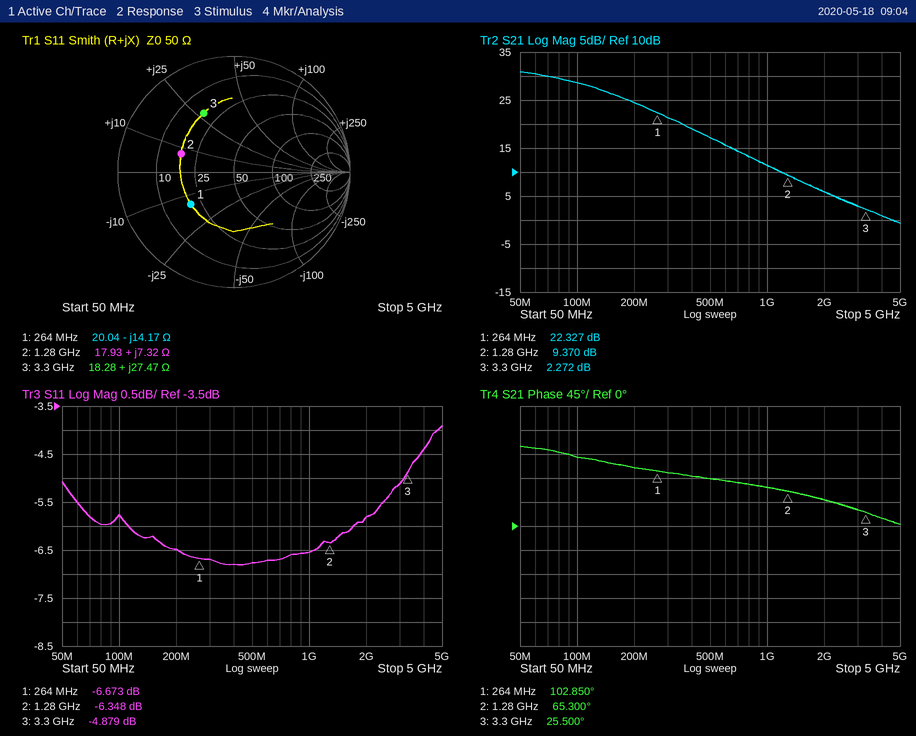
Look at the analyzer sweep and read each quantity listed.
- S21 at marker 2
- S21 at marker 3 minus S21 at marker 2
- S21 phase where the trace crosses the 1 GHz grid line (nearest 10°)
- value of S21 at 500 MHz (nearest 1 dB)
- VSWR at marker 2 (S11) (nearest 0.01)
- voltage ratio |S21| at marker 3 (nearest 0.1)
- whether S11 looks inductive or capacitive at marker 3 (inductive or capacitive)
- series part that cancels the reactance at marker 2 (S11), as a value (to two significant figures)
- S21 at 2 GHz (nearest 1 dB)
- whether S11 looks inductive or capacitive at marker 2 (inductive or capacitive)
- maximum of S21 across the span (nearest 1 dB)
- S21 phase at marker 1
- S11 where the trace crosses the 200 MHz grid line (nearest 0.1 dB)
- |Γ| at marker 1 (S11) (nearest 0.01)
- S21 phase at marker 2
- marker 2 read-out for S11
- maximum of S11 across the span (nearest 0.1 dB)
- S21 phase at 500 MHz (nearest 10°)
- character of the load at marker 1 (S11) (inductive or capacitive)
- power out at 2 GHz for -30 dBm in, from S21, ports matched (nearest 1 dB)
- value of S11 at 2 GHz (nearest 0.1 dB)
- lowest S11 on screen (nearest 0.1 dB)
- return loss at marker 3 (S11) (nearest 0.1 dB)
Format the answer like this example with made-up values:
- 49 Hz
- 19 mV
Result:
- 9.370 dB
- -7.098 dB
- 70°
- 17 dB
- 2.86
- 1.3
- inductive
- 17 pF
- 6 dB
- inductive
- 31 dB
- 102.850°
- -6.5 dB
- 0.46
- 65.300°
- -6.348 dB
- -3.9 dB
- 90°
- capacitive
- -24 dBm
- -5.8 dB
- -6.8 dB
- 4.9 dB
